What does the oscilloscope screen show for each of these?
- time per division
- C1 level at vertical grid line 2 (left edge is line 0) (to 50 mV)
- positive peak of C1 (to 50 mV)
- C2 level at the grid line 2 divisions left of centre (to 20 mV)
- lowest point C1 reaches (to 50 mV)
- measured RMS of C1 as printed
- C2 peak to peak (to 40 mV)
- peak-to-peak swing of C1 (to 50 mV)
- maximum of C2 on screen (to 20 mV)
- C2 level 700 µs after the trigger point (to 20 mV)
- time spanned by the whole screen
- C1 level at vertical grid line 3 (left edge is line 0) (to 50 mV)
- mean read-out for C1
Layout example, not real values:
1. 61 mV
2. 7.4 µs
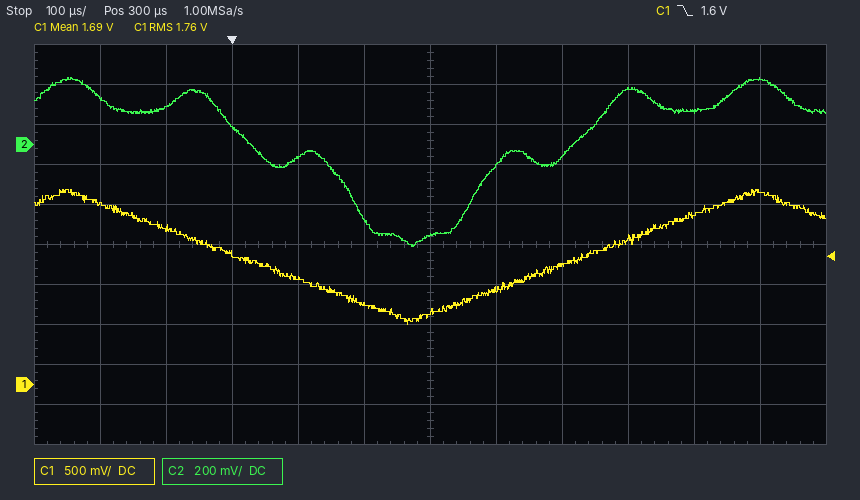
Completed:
1. 100 µs
2. 1.95 V
3. 2.45 V
4. -60 mV
5. 750 mV
6. 1.76 V
7. 840 mV
8. 1.70 V
9. 340 mV
10. 160 mV
11. 1.2 ms
12. 1.65 V
13. 1.69 V
